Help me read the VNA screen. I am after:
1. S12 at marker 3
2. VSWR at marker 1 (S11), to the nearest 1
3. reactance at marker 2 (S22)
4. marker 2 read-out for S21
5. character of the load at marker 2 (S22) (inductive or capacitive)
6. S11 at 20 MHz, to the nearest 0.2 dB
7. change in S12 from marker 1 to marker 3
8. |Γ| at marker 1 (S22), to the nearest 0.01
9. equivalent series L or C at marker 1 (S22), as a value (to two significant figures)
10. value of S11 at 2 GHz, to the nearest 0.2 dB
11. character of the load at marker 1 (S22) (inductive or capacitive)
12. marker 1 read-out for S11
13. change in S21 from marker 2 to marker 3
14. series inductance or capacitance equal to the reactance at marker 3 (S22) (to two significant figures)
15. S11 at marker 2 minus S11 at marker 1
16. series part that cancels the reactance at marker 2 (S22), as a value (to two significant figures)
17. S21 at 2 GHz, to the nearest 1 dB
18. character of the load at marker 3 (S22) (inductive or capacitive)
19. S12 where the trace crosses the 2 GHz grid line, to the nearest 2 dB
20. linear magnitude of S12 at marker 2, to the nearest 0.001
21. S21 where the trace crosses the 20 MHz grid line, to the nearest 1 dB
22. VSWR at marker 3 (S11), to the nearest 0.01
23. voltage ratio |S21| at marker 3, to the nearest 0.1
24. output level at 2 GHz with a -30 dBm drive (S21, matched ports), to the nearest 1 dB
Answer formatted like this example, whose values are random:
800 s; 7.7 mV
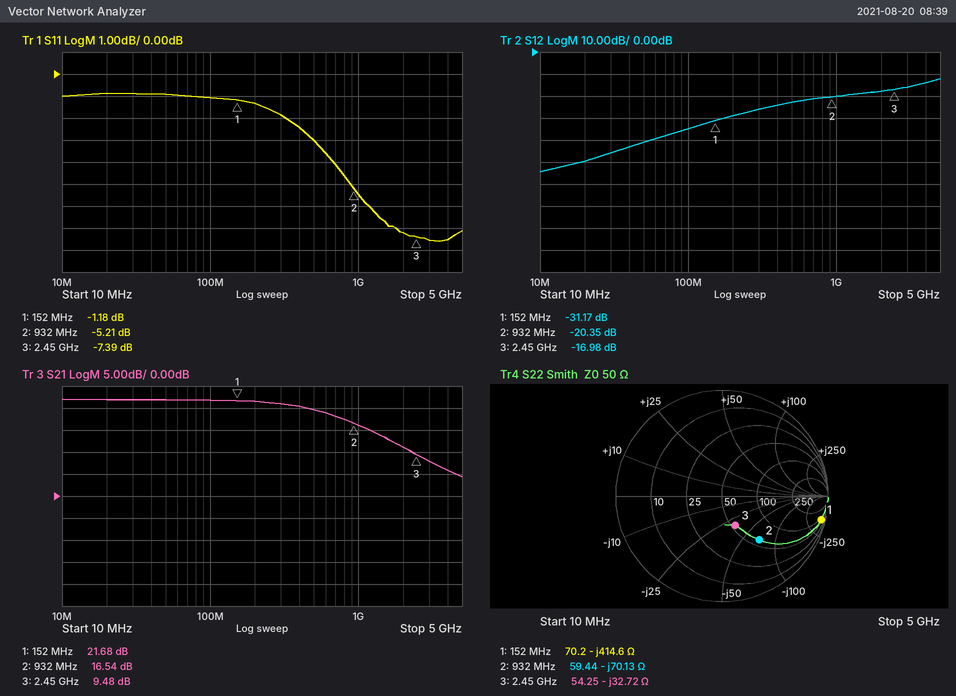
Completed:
-16.98 dB; 15; -70.13 Ω; 16.54 dB; capacitive; -0.8 dB; 14.19 dB; 0.96; 2.5 pF; -7.2 dB; capacitive; -1.18 dB; -7.06 dB; 2.0 pF; -4.03 dB; 12 nH; 11 dB; capacitive; -18 dB; 0.096; 22 dB; 2.49; 3.0; -19 dBm
